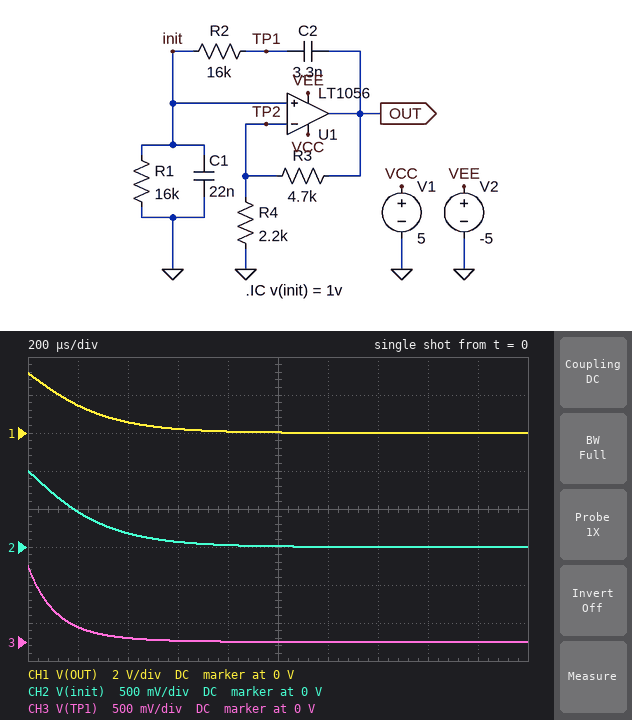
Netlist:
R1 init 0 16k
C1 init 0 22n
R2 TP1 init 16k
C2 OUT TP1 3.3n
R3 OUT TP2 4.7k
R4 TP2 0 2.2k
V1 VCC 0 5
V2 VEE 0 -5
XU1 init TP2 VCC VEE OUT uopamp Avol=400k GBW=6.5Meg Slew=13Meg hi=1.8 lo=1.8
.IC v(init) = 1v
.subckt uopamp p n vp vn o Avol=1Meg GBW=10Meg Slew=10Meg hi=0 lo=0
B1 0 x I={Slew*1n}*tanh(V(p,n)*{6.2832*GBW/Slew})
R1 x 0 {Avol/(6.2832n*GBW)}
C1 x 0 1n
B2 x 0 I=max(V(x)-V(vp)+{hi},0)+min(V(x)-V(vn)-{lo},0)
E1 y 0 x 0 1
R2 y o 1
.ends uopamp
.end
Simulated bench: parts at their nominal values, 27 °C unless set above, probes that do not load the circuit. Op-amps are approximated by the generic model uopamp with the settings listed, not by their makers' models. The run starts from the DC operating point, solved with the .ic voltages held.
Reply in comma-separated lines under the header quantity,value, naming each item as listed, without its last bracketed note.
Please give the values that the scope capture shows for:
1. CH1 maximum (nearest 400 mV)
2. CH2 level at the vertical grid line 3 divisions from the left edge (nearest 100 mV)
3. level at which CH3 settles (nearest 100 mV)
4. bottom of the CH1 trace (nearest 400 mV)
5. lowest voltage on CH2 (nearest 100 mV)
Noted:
quantity,value
CH1 maximum,3.2 V
CH2 level at the vertical grid line 3 divisions from the left edge,100 mV
level at which CH3 settles,0 V
bottom of the CH1 trace,0 V
lowest voltage on CH2,0 V
